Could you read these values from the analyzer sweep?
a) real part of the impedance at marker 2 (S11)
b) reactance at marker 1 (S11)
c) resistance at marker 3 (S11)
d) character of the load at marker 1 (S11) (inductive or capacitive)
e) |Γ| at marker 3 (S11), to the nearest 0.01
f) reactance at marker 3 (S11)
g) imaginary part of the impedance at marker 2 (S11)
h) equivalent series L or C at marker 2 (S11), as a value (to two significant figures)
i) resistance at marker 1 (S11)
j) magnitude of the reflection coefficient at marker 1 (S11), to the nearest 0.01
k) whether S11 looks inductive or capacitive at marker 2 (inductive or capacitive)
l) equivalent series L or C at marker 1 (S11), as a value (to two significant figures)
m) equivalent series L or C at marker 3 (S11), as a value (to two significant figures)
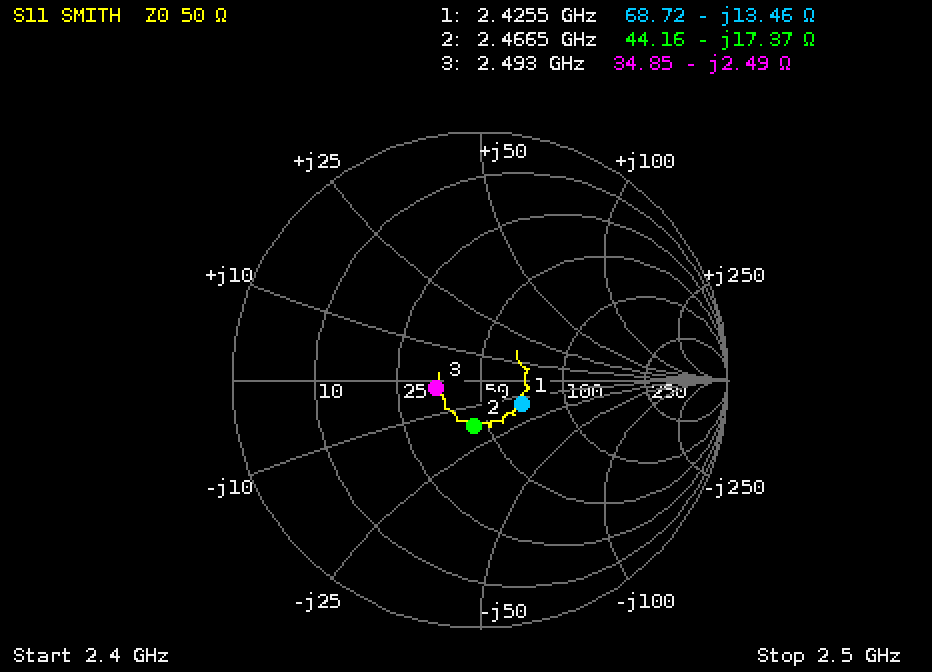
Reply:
44.16 Ω
-13.46 Ω
34.85 Ω
capacitive
0.18
-2.49 Ω
-17.37 Ω
3.7 pF
68.72 Ω
0.19
capacitive
4.9 pF
26 pF
